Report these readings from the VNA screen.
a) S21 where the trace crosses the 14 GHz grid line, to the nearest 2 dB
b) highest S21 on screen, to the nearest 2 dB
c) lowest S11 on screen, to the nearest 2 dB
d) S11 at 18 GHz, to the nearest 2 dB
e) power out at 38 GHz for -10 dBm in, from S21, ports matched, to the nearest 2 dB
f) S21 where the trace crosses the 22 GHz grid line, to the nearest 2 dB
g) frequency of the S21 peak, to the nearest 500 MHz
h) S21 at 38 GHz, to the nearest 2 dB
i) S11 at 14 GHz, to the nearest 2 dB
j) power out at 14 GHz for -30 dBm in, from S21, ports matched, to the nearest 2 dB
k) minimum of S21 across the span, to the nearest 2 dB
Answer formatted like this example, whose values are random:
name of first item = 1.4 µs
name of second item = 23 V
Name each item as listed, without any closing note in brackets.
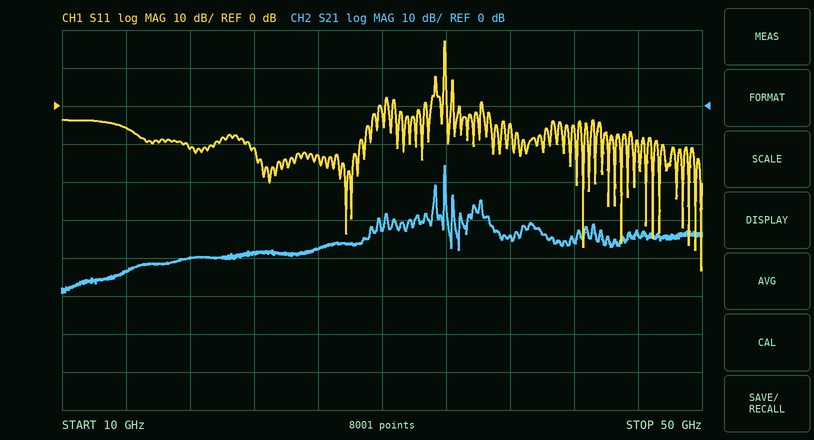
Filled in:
S21 where the trace crosses the 14 GHz grid line, to the nearest 2 dB = -44 dB
highest S21 on screen, to the nearest 2 dB = -16 dB
lowest S11 on screen, to the nearest 2 dB = -44 dB
S11 at 18 GHz, to the nearest 2 dB = -12 dB
power out at 38 GHz for -10 dBm in, from S21, ports matched, to the nearest 2 dB = -44 dBm
S21 where the trace crosses the 22 GHz grid line, to the nearest 2 dB = -38 dB
frequency of the S21 peak, to the nearest 500 MHz = 34.0 GHz
S21 at 38 GHz, to the nearest 2 dB = -34 dB
S11 at 14 GHz, to the nearest 2 dB = -6 dB
power out at 14 GHz for -30 dBm in, from S21, ports matched, to the nearest 2 dB = -74 dBm
minimum of S21 across the span, to the nearest 2 dB = -50 dB
